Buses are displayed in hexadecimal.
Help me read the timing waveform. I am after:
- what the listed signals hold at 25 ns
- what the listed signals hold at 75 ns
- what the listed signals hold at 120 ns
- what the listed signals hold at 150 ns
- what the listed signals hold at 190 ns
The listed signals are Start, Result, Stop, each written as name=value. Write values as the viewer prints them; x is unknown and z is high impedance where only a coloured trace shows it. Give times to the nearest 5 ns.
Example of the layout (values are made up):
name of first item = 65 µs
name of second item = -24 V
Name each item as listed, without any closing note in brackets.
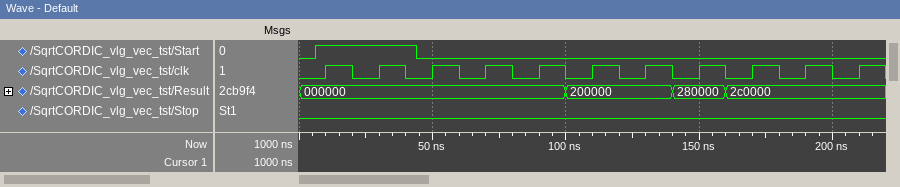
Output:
what the listed signals hold at 25 ns = Start=1, Result=000000, Stop=0
what the listed signals hold at 75 ns = Start=0, Result=000000, Stop=0
what the listed signals hold at 120 ns = Start=0, Result=200000, Stop=0
what the listed signals hold at 150 ns = Start=0, Result=280000, Stop=0
what the listed signals hold at 190 ns = Start=0, Result=2c0000, Stop=0
